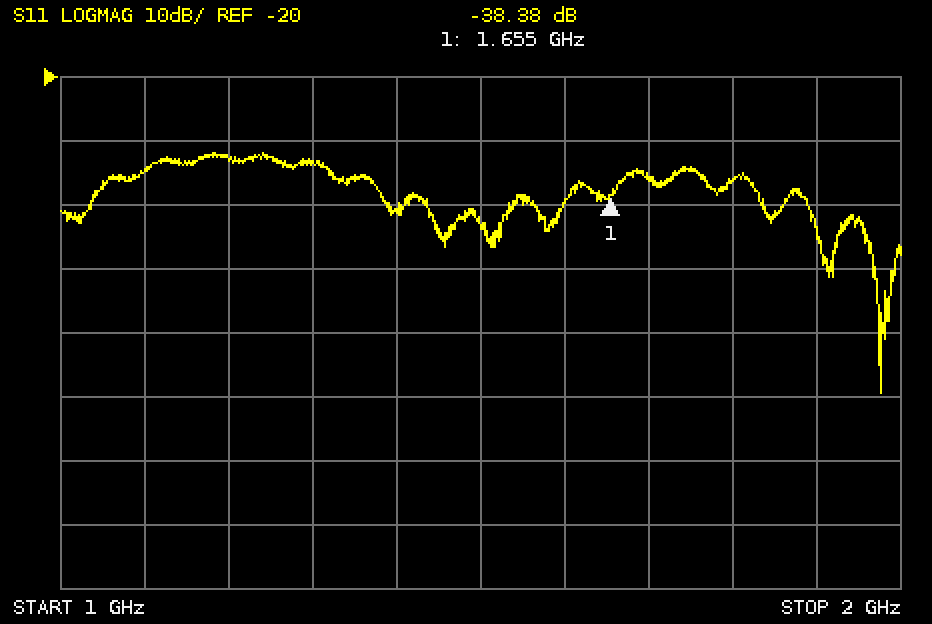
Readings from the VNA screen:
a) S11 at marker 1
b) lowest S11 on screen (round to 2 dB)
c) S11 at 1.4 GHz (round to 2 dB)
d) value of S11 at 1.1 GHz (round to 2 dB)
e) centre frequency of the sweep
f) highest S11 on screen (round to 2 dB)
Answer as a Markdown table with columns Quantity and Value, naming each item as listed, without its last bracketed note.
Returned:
| Quantity | Value |
|---|---|
| S11 at marker 1 | -38.38 dB |
| lowest S11 on screen | -70 dB |
| S11 at 1.4 GHz | -40 dB |
| value of S11 at 1.1 GHz | -34 dB |
| centre frequency of the sweep | 1.5 GHz |
| highest S11 on screen | -32 dB |
